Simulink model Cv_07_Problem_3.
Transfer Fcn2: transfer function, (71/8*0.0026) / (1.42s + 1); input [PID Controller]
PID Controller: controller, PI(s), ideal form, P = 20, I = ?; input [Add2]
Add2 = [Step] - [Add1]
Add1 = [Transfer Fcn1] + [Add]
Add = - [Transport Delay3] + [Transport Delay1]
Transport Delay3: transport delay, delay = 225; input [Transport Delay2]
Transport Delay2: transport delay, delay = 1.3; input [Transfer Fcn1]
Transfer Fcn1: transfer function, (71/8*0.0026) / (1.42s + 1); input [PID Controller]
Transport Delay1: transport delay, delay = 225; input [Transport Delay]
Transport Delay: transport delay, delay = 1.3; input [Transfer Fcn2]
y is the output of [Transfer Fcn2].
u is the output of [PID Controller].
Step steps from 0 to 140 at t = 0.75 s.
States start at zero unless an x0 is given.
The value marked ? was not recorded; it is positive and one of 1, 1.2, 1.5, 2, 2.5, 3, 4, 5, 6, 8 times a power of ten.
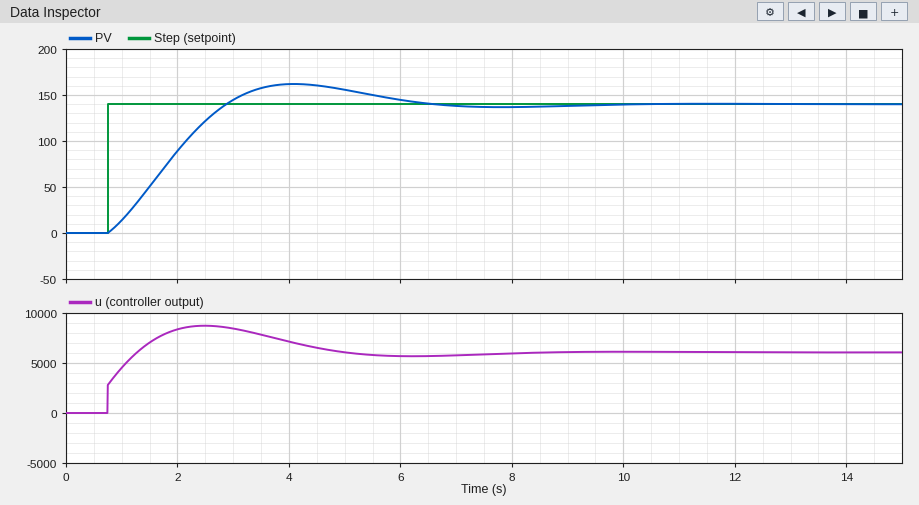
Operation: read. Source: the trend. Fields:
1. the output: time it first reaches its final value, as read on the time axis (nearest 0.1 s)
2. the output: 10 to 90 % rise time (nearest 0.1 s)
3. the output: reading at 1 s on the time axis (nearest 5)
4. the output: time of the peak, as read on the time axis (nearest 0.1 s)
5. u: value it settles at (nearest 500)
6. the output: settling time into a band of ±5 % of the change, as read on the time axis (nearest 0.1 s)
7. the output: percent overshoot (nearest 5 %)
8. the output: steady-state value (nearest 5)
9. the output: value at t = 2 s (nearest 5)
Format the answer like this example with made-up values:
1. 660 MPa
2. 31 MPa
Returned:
1. 2.9 s
2. 1.6 s
3. 15
4. 4.1 s
5. 6000
6. 5.8 s
7. 15 %
8. 140
9. 90
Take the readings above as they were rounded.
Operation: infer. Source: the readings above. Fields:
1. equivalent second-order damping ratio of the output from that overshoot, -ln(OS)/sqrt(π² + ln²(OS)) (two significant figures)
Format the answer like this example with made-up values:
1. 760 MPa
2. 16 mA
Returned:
1. 0.52
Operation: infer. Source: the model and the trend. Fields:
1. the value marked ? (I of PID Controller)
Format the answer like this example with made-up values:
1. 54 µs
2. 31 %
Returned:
1. 3
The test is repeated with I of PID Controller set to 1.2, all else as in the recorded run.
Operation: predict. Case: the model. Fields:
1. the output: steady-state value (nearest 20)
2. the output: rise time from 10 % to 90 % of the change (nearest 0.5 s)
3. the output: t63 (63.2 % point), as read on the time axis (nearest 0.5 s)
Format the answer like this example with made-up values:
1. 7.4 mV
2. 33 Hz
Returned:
1. 140
2. 3.5 s
3. 3.0 s
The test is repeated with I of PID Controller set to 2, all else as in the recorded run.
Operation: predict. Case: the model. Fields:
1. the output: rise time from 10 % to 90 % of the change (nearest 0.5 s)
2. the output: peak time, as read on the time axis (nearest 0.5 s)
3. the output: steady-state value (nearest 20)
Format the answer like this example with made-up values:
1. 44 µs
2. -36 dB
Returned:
1. 2.0 s
2. 5.0 s
3. 140
